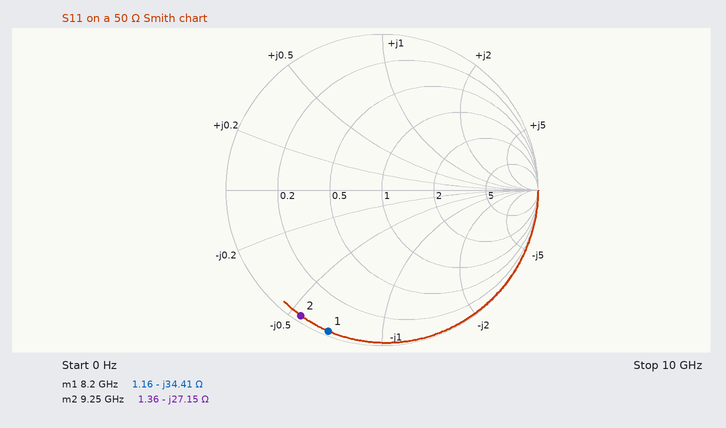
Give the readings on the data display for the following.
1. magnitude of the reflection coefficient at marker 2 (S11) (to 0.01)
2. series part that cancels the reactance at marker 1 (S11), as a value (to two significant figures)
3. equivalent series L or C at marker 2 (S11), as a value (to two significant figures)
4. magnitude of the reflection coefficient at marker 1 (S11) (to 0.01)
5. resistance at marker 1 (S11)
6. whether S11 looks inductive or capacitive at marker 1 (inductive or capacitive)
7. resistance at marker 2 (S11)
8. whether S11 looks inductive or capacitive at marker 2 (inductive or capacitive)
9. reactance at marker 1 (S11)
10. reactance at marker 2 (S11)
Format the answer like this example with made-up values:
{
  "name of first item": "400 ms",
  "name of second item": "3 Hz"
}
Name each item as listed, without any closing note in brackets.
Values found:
{
  "magnitude of the reflection coefficient at marker 2 (S11)": "0.96",
  "series part that cancels the reactance at marker 1 (S11), as a value": "670 pH",
  "equivalent series L or C at marker 2 (S11), as a value": "630 fF",
  "magnitude of the reflection coefficient at marker 1 (S11)": "0.97",
  "resistance at marker 1": "1.16 Ω",
  "whether S11 looks inductive or capacitive at marker 1": "capacitive",
  "resistance at marker 2": "1.36 Ω",
  "whether S11 looks inductive or capacitive at marker 2": "capacitive",
  "reactance at marker 1": "-34.41 Ω",
  "reactance at marker 2": "-27.15 Ω"
}
